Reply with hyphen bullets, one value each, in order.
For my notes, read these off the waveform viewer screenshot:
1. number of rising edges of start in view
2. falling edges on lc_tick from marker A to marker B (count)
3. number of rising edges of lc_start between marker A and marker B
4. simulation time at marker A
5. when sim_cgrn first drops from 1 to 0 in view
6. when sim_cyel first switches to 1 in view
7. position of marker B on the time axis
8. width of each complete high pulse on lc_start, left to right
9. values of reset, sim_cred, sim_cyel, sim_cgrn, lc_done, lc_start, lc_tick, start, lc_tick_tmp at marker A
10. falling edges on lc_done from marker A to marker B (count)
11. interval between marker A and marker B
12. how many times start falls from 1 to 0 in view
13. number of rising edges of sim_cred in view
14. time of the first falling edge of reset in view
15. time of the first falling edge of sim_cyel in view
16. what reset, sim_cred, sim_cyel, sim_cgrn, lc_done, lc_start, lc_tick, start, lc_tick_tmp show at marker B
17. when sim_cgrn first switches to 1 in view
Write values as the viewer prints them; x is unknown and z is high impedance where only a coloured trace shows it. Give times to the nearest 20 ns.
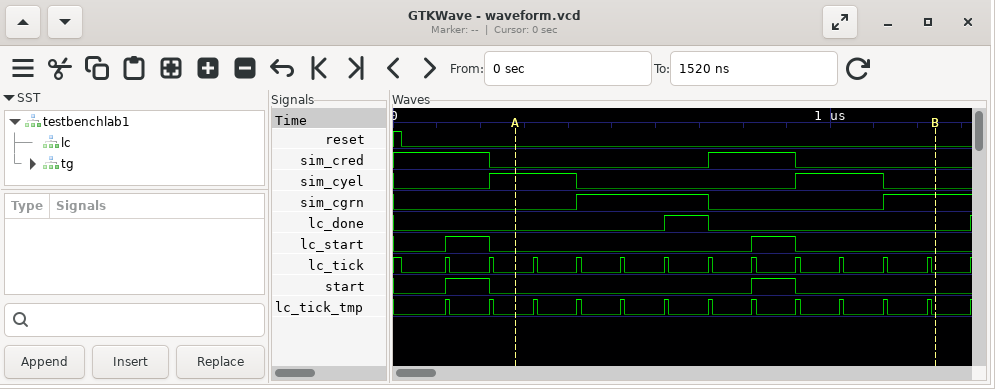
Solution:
- 2
- 10
- 1
- 280 ns
- 720 ns
- 220 ns
- 1240 ns
- 100 ns, 100 ns
- reset=0, sim_cred=0, sim_cyel=1, sim_cgrn=0, lc_done=0, lc_start=0, lc_tick=0, start=0, lc_tick_tmp=0
- 1
- 960 ns
- 2
- 1
- 20 ns
- 420 ns
- reset=0, sim_cred=0, sim_cyel=0, sim_cgrn=1, lc_done=0, lc_start=0, lc_tick=0, start=0, lc_tick_tmp=0
- 420 ns
